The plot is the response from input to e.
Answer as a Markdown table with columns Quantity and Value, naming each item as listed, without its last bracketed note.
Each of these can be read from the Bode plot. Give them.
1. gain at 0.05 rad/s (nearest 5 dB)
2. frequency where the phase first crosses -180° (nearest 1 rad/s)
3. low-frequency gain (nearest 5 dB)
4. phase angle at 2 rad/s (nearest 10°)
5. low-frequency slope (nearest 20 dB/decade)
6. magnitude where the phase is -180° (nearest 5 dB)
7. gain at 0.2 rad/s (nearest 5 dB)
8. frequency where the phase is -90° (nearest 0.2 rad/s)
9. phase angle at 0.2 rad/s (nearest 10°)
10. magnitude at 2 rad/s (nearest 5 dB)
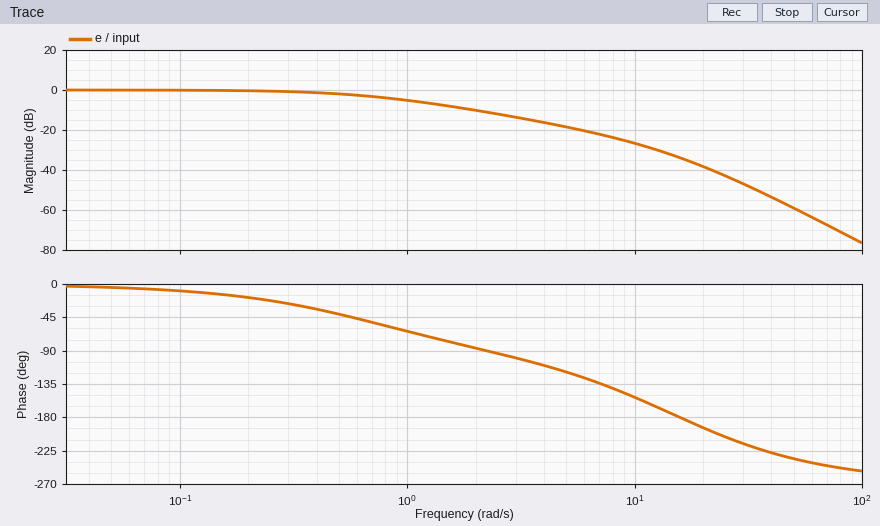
| Quantity | Value |
|---|---|
| gain at 0.05 rad/s | 0 dB |
| frequency where the phase first crosses -180° | 16 rad/s |
| low-frequency gain | 0 dB |
| phase angle at 2 rad/s | -90° |
| low-frequency slope | 0 dB/decade |
| magnitude where the phase is -180° | -35 dB |
| gain at 0.2 rad/s | 0 dB |
| frequency where the phase is -90° | 2.2 rad/s |
| phase angle at 0.2 rad/s | -20° |
| magnitude at 2 rad/s | -10 dB |
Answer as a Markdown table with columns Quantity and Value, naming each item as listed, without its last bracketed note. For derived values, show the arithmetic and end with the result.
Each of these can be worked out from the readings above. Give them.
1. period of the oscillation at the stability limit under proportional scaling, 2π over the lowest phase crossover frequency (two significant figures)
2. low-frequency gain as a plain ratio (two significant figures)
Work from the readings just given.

| Quantity | Value |
|---|---|
| period of the oscillation at the stability limit under proportional scaling, 2π over the lowest phase crossover frequency | 2π / 16 = 0.39 s |
| low-frequency gain as a plain ratio | 10^(0 / 20) = 1.0 |
